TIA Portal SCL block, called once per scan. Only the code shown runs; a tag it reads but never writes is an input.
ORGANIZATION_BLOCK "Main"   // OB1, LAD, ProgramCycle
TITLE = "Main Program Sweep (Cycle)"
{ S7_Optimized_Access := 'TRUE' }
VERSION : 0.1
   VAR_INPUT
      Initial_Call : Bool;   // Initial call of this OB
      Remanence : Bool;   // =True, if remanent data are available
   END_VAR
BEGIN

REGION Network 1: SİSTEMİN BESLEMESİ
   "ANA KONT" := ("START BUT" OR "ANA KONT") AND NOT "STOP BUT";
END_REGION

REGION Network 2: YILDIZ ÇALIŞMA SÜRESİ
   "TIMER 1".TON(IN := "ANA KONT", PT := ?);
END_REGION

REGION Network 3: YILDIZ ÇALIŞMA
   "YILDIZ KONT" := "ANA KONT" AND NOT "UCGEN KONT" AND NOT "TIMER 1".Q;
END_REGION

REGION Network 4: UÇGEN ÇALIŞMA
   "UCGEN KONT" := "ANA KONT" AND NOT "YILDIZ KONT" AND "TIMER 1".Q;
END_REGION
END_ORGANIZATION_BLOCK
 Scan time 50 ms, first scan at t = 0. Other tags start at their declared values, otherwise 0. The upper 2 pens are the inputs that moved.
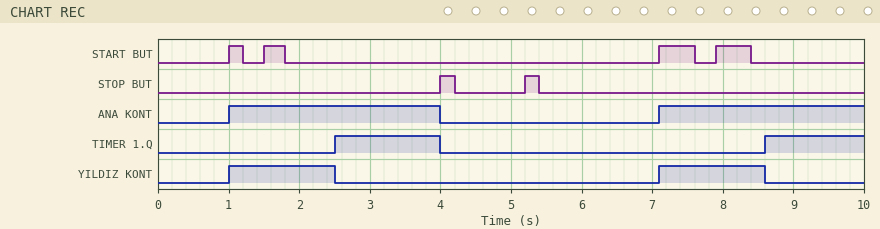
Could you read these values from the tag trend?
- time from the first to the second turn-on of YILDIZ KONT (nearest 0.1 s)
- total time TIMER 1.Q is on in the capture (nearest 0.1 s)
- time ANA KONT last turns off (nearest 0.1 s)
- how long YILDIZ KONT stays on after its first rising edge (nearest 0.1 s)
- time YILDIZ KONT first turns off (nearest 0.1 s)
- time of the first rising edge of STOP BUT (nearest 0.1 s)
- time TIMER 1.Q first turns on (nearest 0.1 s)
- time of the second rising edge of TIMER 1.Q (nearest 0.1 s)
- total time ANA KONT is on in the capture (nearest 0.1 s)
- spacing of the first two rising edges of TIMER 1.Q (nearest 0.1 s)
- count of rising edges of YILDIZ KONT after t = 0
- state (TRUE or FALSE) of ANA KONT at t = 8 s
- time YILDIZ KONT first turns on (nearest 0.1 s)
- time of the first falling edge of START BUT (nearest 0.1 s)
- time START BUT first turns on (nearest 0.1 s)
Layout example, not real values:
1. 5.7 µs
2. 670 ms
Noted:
1. 6.1 s
2. 2.9 s
3. 4.0 s
4. 1.5 s
5. 2.5 s
6. 4.0 s
7. 2.5 s
8. 8.6 s
9. 5.9 s
10. 6.1 s
11. 2
12. TRUE
13. 1.0 s
14. 1.2 s
15. 1.0 s
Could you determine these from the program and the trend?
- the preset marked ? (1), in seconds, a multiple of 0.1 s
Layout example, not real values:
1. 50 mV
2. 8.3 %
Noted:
1. 1.5 s
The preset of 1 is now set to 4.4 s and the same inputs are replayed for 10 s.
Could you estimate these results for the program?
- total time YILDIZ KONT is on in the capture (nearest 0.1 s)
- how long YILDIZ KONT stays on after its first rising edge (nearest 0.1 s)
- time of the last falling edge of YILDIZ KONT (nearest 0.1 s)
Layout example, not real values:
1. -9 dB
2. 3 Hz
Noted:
1. 5.9 s
2. 3.0 s
3. 4.0 s
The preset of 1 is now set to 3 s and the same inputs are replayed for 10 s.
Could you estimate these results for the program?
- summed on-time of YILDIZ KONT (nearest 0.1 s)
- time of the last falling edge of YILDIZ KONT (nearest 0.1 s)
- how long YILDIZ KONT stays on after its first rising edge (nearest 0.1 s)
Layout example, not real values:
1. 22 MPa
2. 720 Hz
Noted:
1. 5.9 s
2. 4.0 s
3. 3.0 s
